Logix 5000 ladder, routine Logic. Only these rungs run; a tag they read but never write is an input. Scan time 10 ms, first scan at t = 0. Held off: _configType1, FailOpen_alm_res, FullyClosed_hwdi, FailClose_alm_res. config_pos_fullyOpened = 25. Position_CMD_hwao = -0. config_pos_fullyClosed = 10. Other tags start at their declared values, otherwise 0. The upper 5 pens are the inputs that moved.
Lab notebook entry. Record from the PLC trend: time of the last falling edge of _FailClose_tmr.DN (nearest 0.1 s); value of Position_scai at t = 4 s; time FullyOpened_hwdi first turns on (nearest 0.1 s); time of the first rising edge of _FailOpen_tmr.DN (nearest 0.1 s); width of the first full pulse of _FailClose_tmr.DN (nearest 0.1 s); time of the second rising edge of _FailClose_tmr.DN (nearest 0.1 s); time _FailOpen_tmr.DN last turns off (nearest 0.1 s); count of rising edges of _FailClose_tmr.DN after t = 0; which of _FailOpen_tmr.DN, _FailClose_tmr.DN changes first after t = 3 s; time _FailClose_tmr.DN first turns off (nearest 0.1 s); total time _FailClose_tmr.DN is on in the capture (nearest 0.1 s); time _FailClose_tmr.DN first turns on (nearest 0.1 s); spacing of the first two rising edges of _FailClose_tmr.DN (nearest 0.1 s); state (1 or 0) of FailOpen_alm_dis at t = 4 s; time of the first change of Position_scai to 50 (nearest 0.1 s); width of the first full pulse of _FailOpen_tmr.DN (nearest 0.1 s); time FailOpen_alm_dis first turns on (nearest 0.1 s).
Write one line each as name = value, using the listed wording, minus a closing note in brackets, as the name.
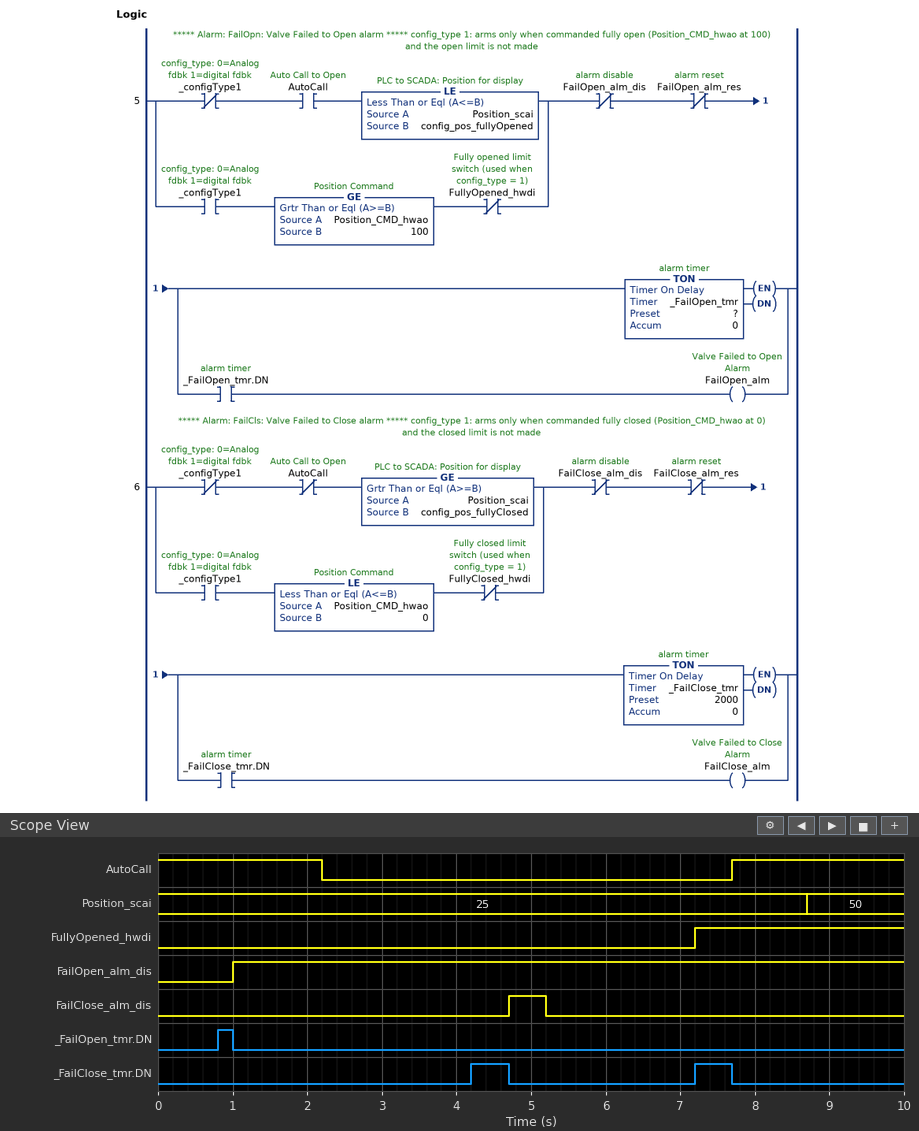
time of the last falling edge of _FailClose_tmr.DN = 7.7 s
value of Position_scai at t = 4 s = 25
time FullyOpened_hwdi first turns on = 7.2 s
time of the first rising edge of _FailOpen_tmr.DN = 0.8 s
width of the first full pulse of _FailClose_tmr.DN = 0.5 s
time of the second rising edge of _FailClose_tmr.DN = 7.2 s
time _FailOpen_tmr.DN last turns off = 1.0 s
count of rising edges of _FailClose_tmr.DN after t = 0 = 2
which of _FailOpen_tmr.DN, _FailClose_tmr.DN changes first after t = 3 s = _FailClose_tmr.DN
time _FailClose_tmr.DN first turns off = 4.7 s
total time _FailClose_tmr.DN is on in the capture = 1.0 s
time _FailClose_tmr.DN first turns on = 4.2 s
spacing of the first two rising edges of _FailClose_tmr.DN = 3.0 s
state (1 or 0) of FailOpen_alm_dis at t = 4 s = 1
time of the first change of Position_scai to 50 = 8.7 s
width of the first full pulse of _FailOpen_tmr.DN = 0.2 s
time FailOpen_alm_dis first turns on = 1.0 s
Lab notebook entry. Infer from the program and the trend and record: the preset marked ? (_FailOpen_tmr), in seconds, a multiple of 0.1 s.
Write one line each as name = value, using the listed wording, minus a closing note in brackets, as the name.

the preset marked ? (_FailOpen_tmr), in seconds, a multiple of 0.1 s = 0.8 s
